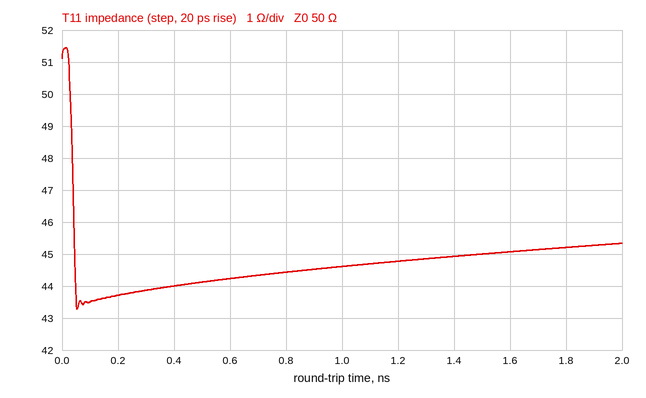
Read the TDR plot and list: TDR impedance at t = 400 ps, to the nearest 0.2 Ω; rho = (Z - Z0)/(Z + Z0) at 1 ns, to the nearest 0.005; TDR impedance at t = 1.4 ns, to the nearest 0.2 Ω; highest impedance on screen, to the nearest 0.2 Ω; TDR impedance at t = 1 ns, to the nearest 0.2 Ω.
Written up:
44.0 Ω
-0.055
45.0 Ω
51.4 Ω
44.6 Ω
